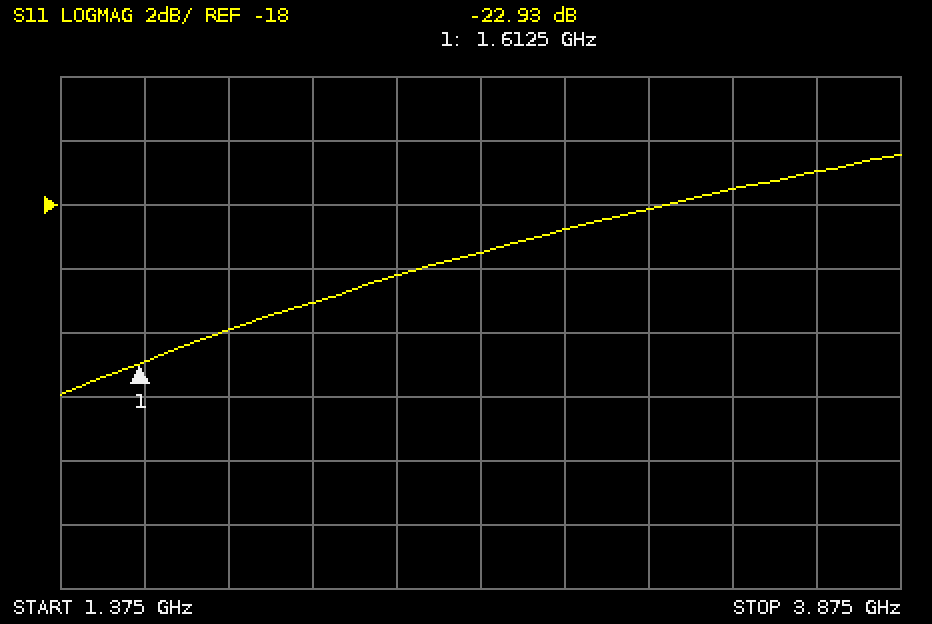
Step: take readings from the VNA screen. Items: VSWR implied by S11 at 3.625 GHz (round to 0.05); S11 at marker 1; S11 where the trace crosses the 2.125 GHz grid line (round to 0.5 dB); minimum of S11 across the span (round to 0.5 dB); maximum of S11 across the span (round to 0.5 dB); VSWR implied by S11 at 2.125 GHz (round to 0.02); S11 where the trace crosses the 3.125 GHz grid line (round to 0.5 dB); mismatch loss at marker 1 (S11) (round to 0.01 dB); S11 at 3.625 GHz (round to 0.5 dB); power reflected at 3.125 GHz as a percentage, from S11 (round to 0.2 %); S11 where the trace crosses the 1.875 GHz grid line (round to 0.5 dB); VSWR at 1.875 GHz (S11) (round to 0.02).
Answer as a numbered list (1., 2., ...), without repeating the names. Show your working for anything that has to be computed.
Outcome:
1. |Γ| = 10^(-17/20) = 0.1413; VSWR = (1 + 0.1413)/(1 − 0.1413) ≈ 1.33, so 1.35 to the nearest 0.05
2. -22.93 dB
3. -21.0 dB
4. -24.0 dB
5. -16.5 dB
6. |Γ| = 10^(-21/20) = 0.0891; VSWR = (1 + 0.0891)/(1 − 0.0891) ≈ 1.20
7. -18.0 dB
8. −10 log10(1 − 10^(-22.93/10)) ≈ 0.02 dB
9. -17.0 dB
10. 10^(-18/10) ≈ 1.6 %
11. -22.0 dB
12. |Γ| = 10^(-22/20) = 0.0794; VSWR = (1 + 0.0794)/(1 − 0.0794) ≈ 1.17, so 1.18 to the nearest 0.02
